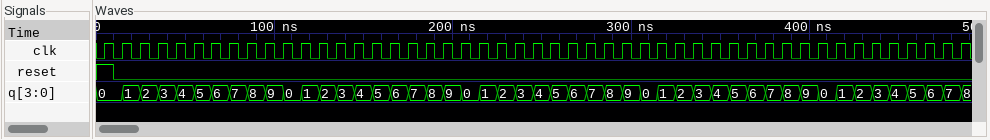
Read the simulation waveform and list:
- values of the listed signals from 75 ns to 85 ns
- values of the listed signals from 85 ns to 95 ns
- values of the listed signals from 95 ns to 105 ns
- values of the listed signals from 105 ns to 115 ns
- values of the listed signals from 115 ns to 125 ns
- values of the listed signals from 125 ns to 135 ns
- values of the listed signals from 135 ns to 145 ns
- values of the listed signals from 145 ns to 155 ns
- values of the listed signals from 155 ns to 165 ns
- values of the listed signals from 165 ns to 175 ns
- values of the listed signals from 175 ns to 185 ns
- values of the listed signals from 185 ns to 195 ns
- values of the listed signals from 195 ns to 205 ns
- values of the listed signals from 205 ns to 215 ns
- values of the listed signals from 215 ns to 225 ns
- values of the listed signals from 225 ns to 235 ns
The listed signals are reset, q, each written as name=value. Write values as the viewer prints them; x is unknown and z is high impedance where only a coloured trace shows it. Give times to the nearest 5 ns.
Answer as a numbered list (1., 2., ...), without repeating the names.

1. reset=0, q=7
2. reset=0, q=8
3. reset=0, q=9
4. reset=0, q=0
5. reset=0, q=1
6. reset=0, q=2
7. reset=0, q=3
8. reset=0, q=4
9. reset=0, q=5
10. reset=0, q=6
11. reset=0, q=7
12. reset=0, q=8
13. reset=0, q=9
14. reset=0, q=0
15. reset=0, q=1
16. reset=0, q=2
